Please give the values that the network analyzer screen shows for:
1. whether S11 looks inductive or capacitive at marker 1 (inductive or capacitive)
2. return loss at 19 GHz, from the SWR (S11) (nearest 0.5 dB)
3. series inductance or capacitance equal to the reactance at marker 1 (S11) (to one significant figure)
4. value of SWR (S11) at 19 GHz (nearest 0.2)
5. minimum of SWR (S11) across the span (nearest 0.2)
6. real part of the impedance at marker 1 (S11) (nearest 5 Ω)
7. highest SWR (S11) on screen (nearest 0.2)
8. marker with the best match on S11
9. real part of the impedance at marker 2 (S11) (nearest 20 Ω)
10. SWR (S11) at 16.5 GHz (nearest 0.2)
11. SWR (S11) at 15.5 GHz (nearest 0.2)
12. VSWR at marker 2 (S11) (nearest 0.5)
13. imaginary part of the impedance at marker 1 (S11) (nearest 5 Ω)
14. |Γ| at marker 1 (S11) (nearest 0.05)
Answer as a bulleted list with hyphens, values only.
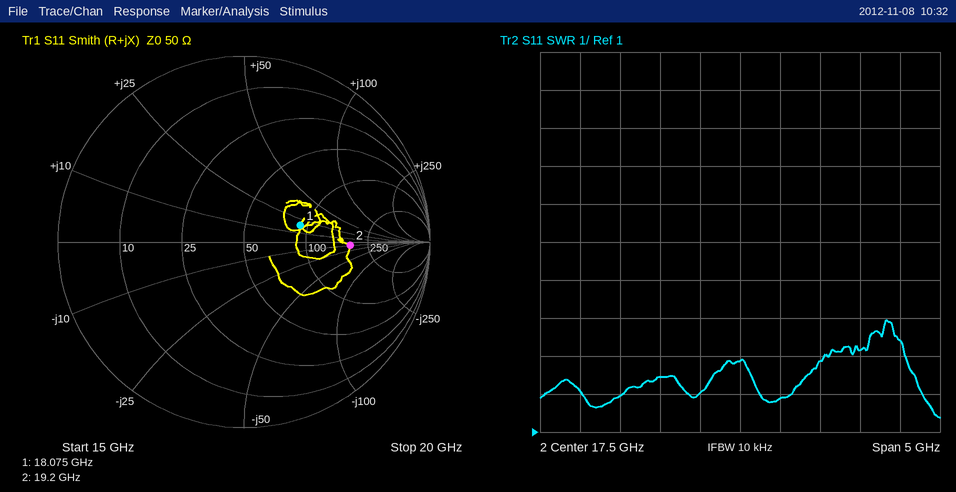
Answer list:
- inductive
- 5.5 dB
- 200 pH
- 3.2
- 1.4
- 90 Ω
- 4.0
- marker 1
- 180 Ω
- 2.4
- 2.0
- 3.5
- +20 Ω
- 0.30
